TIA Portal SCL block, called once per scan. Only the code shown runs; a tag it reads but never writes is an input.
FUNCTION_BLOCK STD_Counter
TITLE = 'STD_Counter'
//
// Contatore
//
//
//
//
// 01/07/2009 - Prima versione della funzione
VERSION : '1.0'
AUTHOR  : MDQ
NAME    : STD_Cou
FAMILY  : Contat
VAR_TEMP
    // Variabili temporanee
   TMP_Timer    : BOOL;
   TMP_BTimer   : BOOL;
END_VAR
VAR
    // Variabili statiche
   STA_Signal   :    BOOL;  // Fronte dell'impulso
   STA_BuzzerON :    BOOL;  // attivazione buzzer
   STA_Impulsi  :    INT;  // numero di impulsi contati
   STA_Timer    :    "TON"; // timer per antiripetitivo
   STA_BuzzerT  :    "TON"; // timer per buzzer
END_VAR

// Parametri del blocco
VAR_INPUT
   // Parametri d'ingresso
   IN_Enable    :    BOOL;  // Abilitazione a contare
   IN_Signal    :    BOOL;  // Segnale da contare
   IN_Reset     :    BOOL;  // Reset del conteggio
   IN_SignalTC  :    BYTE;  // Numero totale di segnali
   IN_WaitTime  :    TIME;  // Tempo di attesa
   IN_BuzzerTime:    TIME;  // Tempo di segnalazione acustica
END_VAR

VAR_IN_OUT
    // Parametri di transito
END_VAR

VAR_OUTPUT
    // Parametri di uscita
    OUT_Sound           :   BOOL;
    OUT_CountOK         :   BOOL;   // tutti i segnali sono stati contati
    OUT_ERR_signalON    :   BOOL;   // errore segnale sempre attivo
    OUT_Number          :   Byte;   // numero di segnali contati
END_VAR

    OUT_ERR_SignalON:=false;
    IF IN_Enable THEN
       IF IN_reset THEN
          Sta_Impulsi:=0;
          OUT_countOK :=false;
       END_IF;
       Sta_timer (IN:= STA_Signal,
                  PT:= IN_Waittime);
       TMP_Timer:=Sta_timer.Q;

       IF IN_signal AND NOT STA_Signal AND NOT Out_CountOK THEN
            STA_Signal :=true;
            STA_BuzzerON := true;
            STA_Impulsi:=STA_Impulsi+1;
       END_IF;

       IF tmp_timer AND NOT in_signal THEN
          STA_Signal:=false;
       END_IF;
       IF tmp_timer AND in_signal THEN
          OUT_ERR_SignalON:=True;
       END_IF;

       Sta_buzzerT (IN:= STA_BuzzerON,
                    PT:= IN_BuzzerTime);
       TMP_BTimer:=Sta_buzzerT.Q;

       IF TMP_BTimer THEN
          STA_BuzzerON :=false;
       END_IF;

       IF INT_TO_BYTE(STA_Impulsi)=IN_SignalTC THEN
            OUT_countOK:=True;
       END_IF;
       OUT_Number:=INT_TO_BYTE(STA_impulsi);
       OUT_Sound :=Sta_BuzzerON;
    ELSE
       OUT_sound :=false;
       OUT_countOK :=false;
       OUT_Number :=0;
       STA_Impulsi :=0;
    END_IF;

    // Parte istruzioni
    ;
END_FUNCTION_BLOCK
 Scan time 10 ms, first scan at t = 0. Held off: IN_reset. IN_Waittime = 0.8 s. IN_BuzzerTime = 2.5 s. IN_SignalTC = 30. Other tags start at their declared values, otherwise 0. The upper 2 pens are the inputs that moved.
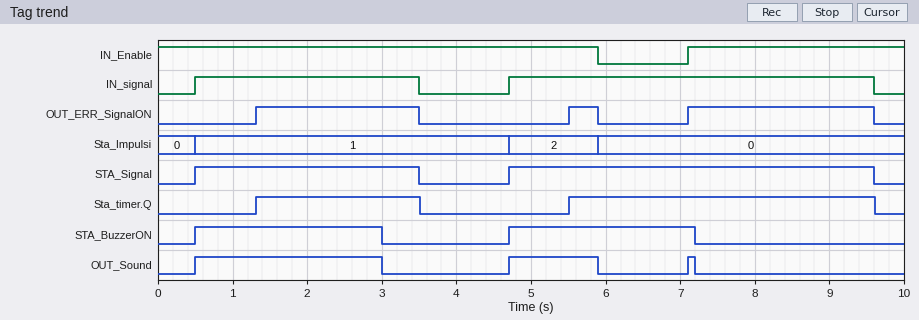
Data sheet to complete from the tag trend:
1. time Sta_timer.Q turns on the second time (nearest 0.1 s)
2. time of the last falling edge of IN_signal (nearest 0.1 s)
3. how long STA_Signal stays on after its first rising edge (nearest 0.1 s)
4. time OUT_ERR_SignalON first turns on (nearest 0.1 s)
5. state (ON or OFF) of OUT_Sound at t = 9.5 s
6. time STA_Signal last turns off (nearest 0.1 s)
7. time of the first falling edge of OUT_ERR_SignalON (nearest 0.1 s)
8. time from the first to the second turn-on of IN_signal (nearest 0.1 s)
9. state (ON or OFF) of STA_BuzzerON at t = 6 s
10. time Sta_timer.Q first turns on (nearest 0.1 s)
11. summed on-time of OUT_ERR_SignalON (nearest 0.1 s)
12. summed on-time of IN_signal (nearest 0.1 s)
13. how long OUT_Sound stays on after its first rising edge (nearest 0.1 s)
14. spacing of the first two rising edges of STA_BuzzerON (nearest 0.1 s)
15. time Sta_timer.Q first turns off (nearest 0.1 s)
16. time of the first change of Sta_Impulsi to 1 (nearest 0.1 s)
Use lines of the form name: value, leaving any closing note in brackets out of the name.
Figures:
time Sta_timer.Q turns on the second time: 5.5 s
time of the last falling edge of IN_signal: 9.6 s
how long STA_Signal stays on after its first rising edge: 3.0 s
time OUT_ERR_SignalON first turns on: 1.3 s
state (ON or OFF) of OUT_Sound at t = 9.5 s: OFF
time STA_Signal last turns off: 9.6 s
time of the first falling edge of OUT_ERR_SignalON: 3.5 s
time from the first to the second turn-on of IN_signal: 4.2 s
state (ON or OFF) of STA_BuzzerON at t = 6 s: ON
time Sta_timer.Q first turns on: 1.3 s
summed on-time of OUT_ERR_SignalON: 5.1 s
summed on-time of IN_signal: 7.9 s
how long OUT_Sound stays on after its first rising edge: 2.5 s
spacing of the first two rising edges of STA_BuzzerON: 4.2 s
time Sta_timer.Q first turns off: 3.5 s
time of the first change of Sta_Impulsi to 1: 0.5 s
